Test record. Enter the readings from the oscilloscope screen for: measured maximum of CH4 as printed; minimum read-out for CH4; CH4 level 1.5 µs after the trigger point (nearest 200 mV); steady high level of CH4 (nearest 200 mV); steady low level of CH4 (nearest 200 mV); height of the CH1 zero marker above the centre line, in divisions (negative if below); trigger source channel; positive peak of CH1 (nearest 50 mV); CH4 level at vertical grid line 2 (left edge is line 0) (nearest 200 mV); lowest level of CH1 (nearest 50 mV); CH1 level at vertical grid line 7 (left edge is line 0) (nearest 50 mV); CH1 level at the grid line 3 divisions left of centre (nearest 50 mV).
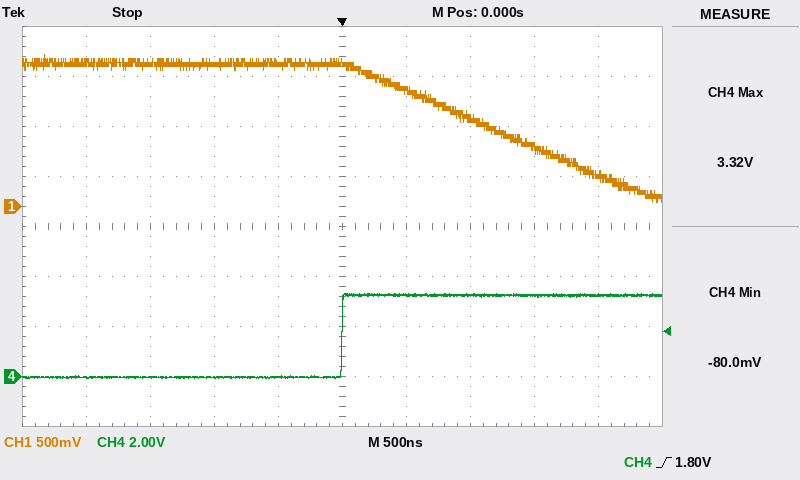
3.32 V
-80.0 mV
3.2 V
3.2 V
0.0 V
+0.4 div
CH4
1.50 V
0.0 V
50 mV
900 mV
1.45 V
